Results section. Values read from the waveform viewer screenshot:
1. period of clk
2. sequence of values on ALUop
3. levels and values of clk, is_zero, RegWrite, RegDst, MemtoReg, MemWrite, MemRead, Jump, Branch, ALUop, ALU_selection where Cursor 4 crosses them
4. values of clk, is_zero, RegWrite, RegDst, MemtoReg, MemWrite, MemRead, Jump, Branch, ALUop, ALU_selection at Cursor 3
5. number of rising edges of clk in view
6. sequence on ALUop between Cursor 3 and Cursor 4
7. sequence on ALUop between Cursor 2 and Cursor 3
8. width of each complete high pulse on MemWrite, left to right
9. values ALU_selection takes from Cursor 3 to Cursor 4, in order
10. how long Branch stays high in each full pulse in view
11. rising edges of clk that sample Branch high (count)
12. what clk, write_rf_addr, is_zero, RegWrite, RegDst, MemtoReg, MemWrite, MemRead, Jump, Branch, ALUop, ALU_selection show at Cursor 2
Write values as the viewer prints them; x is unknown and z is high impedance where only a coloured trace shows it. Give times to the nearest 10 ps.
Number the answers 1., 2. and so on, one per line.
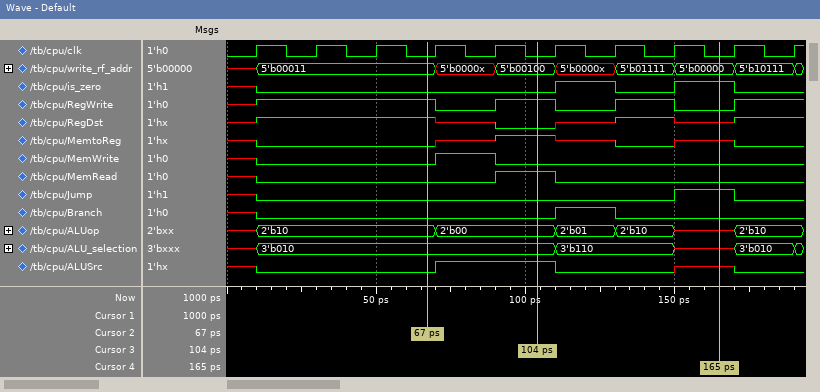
1. 20 ps
2. x, 2'b10, 2'b00, 2'b01, 2'b10, x, 2'b10
3. clk=0, is_zero=1, RegWrite=0, RegDst=x, MemtoReg=x, MemWrite=0, MemRead=0, Jump=1, Branch=0, ALUop=x, ALU_selection=x
4. clk=0, is_zero=0, RegWrite=1, RegDst=0, MemtoReg=1, MemWrite=0, MemRead=1, Jump=0, Branch=0, ALUop=2'b00, ALU_selection=3'b010
5. 10
6. 2'b00, 2'b01, 2'b10, x
7. 2'b10, 2'b00
8. 20 ps
9. 3'b010, 3'b110, x
10. 20 ps
11. 1
12. clk=0, write_rf_addr=5'b00011, is_zero=0, RegWrite=1, RegDst=1, MemtoReg=0, MemWrite=0, MemRead=0, Jump=0, Branch=0, ALUop=2'b10, ALU_selection=3'b010
